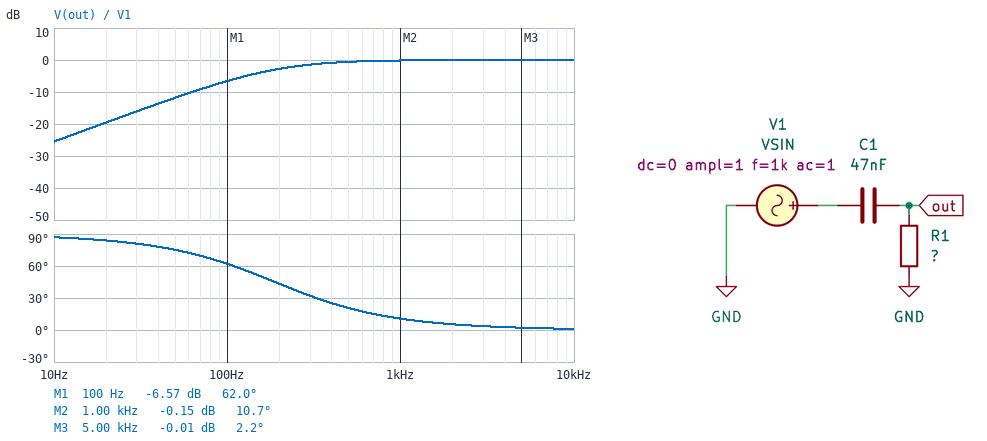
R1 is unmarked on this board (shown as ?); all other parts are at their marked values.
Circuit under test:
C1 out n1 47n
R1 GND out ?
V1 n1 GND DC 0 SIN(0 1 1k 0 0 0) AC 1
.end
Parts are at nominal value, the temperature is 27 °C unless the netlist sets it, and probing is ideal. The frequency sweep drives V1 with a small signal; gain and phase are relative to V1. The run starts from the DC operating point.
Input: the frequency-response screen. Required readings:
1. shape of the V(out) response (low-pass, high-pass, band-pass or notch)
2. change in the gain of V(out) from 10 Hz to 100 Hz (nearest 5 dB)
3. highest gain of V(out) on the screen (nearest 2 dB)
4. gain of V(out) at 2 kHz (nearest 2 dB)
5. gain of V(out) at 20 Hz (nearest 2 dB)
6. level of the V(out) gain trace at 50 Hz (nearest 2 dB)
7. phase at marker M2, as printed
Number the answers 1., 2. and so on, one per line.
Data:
1. high-pass
2. 20 dB
3. 0 dB
4. 0 dB
5. -20 dB
6. -12 dB
7. 10.7 deg
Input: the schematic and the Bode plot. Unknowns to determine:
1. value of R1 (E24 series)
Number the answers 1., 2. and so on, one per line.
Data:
1. 18 kΩ
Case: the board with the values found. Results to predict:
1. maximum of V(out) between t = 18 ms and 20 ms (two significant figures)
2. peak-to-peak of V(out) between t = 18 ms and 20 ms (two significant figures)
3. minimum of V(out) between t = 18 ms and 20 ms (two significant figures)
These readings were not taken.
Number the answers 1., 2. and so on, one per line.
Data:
1. 980 mV
2. 2.0 V
3. -980 mV
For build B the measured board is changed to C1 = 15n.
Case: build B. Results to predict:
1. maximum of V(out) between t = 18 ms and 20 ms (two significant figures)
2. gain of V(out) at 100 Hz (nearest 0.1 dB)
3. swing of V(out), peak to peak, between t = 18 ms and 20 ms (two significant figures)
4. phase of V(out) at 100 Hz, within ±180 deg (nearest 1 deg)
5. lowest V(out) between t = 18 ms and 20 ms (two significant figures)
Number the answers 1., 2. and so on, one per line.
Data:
1. 860 mV
2. -15.5 dB
3. 1.7 V
4. 80 deg
5. -860 mV
